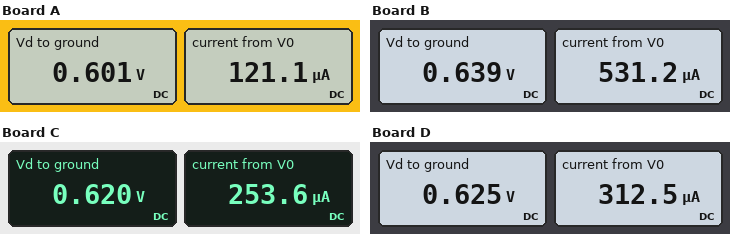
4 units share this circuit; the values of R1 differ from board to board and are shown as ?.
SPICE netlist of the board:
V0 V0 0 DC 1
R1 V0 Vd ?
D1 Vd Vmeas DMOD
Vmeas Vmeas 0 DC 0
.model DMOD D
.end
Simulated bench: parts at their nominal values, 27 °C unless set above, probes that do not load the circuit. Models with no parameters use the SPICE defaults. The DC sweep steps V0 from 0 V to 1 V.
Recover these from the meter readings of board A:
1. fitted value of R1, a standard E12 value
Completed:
3.3 kΩ
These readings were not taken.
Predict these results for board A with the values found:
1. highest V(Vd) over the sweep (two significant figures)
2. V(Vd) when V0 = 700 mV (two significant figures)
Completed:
600 mV
570 mV
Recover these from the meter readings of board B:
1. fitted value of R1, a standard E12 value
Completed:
680 Ω
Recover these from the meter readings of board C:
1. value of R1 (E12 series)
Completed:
1.5 kΩ
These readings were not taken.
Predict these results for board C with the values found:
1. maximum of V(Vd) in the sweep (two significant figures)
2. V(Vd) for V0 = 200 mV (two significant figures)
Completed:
620 mV
200 mV
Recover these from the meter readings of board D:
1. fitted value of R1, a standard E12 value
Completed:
1.2 kΩ
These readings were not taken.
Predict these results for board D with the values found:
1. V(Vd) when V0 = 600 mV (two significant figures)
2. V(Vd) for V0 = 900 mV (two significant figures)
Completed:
560 mV
620 mV
